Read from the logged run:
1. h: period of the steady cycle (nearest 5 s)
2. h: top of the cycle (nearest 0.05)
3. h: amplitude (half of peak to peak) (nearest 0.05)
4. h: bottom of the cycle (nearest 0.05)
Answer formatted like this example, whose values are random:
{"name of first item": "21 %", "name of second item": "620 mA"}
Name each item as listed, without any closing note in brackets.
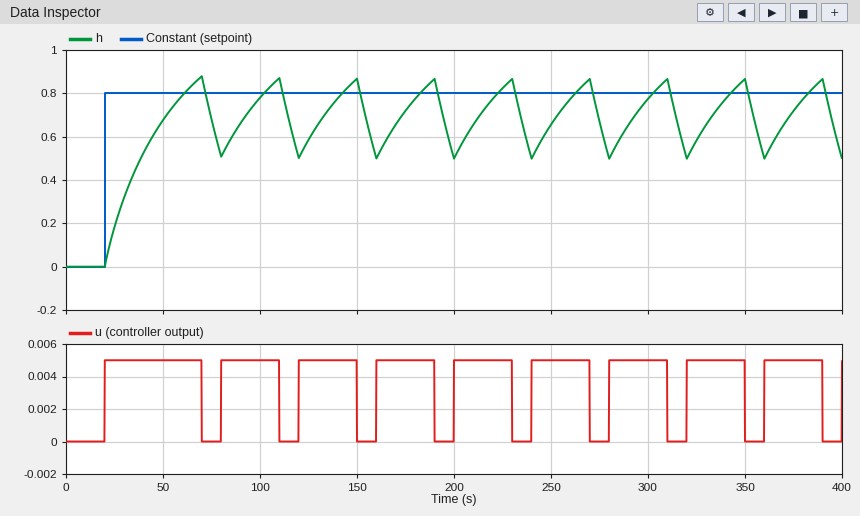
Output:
{"h: period of the steady cycle": "40 s", "h: top of the cycle": "0.85", "h: amplitude (half of peak to peak)": "0.20", "h: bottom of the cycle": "0.50"}
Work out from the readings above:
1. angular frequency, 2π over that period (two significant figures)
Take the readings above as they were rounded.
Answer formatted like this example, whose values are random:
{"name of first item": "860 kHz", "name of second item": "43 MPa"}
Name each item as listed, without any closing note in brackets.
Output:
{"angular frequency, 2π over that period": "0.16 rad/s"}
